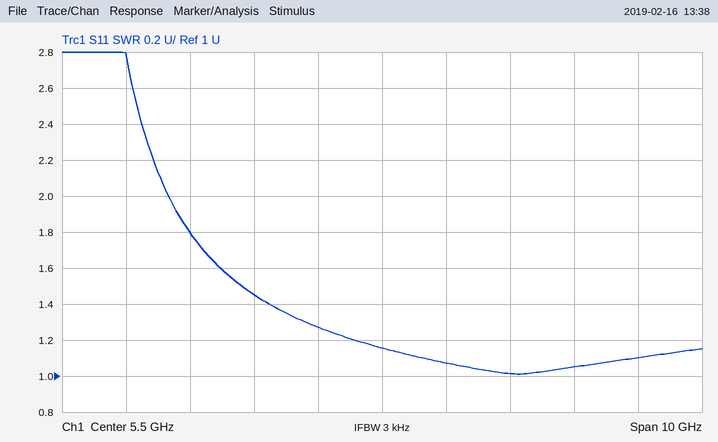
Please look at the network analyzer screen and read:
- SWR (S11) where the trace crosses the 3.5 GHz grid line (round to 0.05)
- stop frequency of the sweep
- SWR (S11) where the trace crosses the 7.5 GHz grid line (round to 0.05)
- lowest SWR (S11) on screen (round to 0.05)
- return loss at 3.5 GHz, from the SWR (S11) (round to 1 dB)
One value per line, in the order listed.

1.45
10.5 GHz
1.00
1.00
15 dB
